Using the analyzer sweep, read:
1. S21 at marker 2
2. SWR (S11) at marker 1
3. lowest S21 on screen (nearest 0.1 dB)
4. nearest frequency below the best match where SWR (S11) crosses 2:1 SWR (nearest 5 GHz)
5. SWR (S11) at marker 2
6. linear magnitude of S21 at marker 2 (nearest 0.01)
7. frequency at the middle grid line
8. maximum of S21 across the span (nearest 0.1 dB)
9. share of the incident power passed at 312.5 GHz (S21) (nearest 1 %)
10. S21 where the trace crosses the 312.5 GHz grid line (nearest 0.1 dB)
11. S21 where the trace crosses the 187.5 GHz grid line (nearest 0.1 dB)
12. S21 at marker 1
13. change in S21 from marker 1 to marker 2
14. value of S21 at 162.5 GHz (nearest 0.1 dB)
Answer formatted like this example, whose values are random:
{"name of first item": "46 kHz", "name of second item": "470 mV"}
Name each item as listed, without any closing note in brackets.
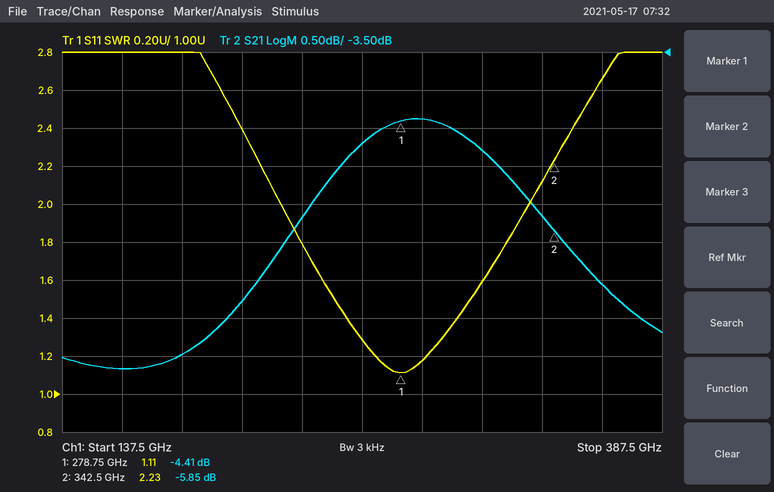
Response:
{"S21 at marker 2": "-5.85 dB", "SWR (S11) at marker 1": "1.11", "lowest S21 on screen": "-7.7 dB", "nearest frequency below the best match where SWR (S11) crosses 2:1 SWR": "230 GHz", "SWR (S11) at marker 2": "2.23", "linear magnitude of S21 at marker 2": "0.51", "frequency at the middle grid line": "262.5 GHz", "maximum of S21 across the span": "-4.4 dB", "share of the incident power passed at 312.5 GHz (S21)": "33 %", "S21 where the trace crosses the 312.5 GHz grid line": "-4.8 dB", "S21 where the trace crosses the 187.5 GHz grid line": "-7.5 dB", "S21 at marker 1": "-4.41 dB", "change in S21 from marker 1 to marker 2": "-1.44 dB", "value of S21 at 162.5 GHz": "-7.7 dB"}
